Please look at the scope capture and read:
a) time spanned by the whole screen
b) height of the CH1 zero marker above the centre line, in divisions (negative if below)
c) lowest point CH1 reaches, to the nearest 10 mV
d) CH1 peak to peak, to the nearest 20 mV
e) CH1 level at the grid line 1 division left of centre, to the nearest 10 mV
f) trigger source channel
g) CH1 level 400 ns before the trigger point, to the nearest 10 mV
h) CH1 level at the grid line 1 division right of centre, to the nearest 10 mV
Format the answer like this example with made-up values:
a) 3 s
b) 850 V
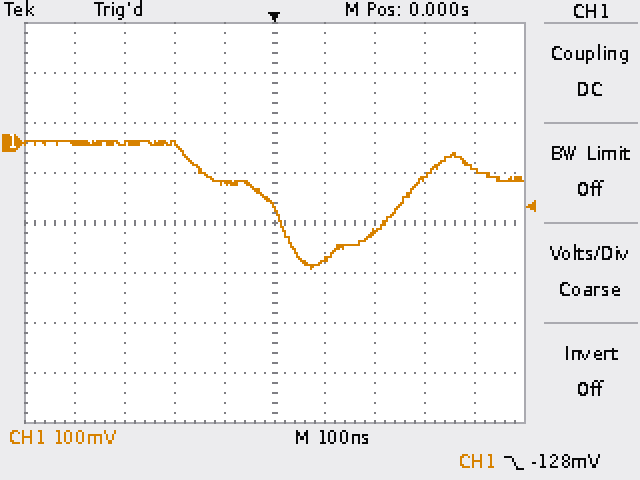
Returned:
a) 1 µs
b) +1.6 div
c) -250 mV
d) 260 mV
e) -80 mV
f) CH1
g) 0 mV
h) -230 mV
